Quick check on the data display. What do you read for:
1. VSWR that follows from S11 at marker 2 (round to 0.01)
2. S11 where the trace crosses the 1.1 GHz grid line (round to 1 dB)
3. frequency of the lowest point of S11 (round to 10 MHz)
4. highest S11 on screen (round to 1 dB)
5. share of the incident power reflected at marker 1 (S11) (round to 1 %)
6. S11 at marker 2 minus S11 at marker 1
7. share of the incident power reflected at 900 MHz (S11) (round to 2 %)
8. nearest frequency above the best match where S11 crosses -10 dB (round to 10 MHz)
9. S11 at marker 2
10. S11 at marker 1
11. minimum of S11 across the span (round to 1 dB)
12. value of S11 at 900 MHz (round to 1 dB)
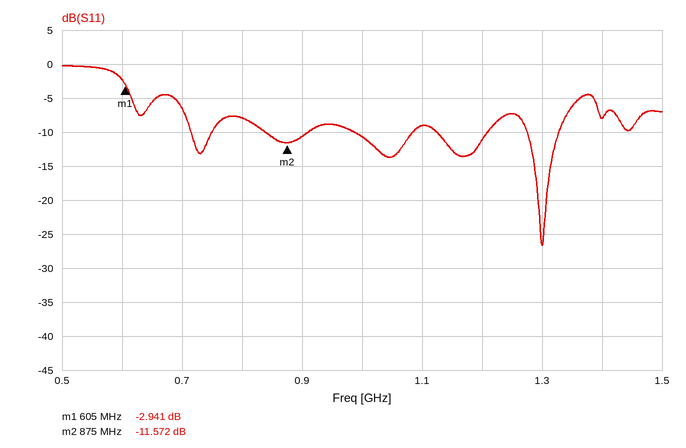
1.72
-9 dB
1.30 GHz
0 dB
51 %
-8.631 dB
8 %
1.33 GHz
-11.572 dB
-2.941 dB
-27 dB
-11 dB
